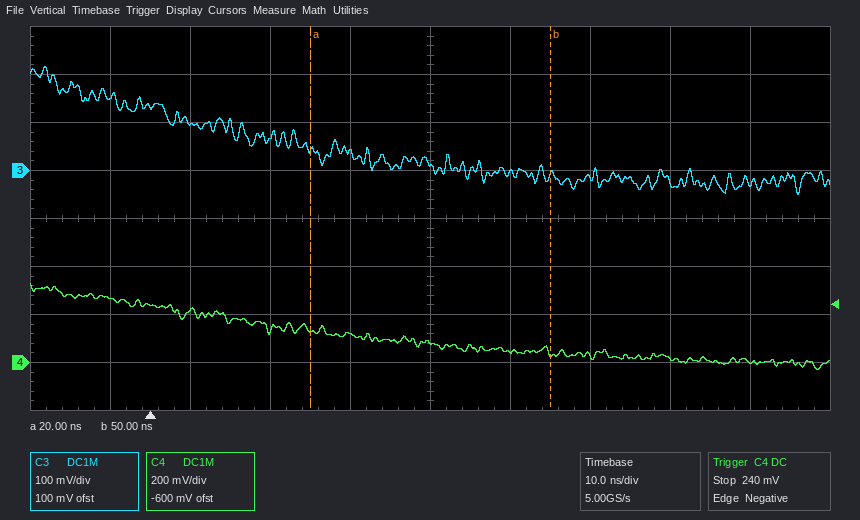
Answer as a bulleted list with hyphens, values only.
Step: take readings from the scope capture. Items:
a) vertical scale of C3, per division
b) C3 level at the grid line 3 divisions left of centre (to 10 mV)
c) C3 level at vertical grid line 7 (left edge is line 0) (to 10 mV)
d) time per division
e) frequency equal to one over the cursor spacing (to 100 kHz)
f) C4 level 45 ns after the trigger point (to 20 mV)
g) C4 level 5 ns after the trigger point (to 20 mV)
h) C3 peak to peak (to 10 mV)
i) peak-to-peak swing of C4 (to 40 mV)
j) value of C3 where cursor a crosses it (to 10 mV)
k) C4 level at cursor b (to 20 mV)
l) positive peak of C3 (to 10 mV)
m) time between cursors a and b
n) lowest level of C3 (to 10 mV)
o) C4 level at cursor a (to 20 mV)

- 100 mV
- 100 mV
- -10 mV
- 10 ns
- 33.3 MHz
- 40 mV
- 220 mV
- 270 mV
- 360 mV
- 40 mV
- 40 mV
- 220 mV
- 30 ns
- -50 mV
- 140 mV
